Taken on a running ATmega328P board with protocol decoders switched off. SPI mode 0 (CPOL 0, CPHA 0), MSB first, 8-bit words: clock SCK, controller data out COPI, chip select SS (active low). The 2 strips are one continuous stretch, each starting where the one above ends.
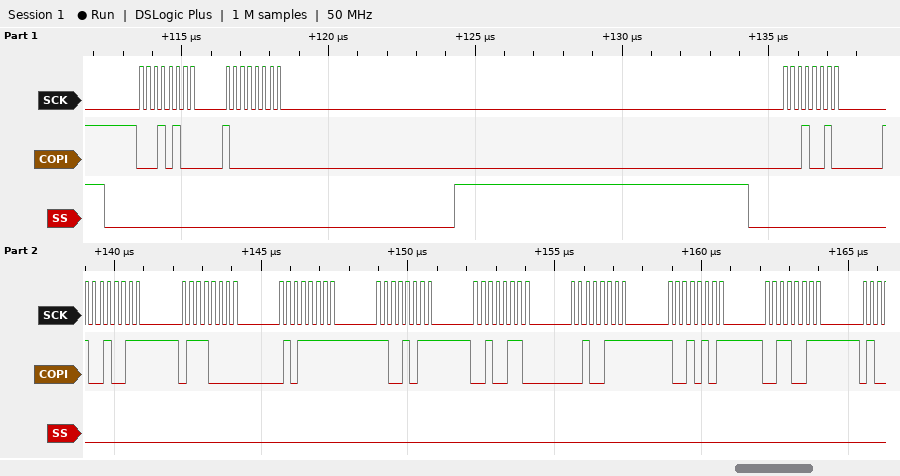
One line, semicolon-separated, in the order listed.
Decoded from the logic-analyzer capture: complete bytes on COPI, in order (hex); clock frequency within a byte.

14 80 12 93 70 5F CB 26 27 95 33; 4 MHz
